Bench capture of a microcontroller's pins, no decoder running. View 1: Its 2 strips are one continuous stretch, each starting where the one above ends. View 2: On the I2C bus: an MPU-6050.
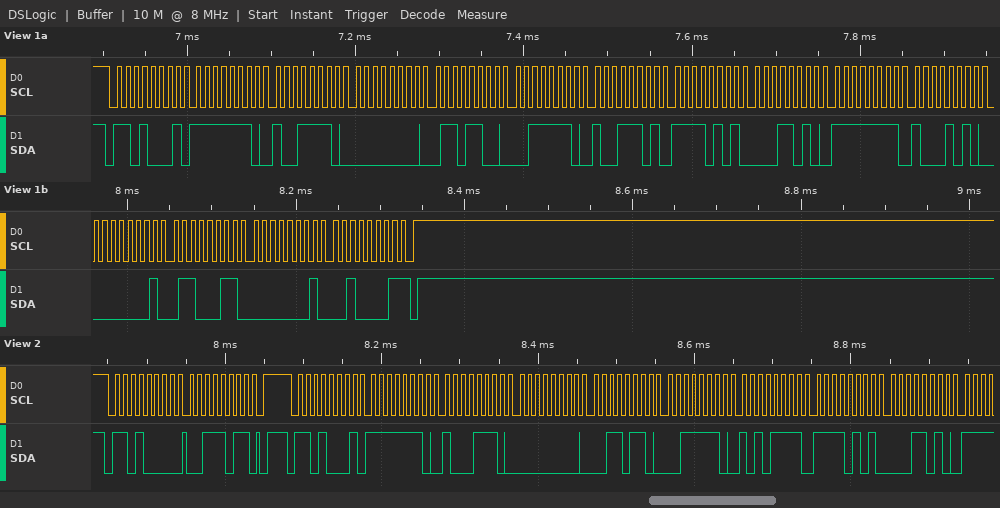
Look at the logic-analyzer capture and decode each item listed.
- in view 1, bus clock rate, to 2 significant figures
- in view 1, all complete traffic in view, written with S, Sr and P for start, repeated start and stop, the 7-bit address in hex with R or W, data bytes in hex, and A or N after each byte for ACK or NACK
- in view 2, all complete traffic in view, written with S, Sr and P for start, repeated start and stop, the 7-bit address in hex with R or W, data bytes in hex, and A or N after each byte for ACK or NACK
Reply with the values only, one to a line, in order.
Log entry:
100 kHz
S 68R A FE A 9E A 00 A 6C A 3E A 9D A F5 A 1A A FF A 8A A 01 A 63 A 01 A 21 N P
S 68W A 3B A P S 68R A FE A 8E A 00 A 36 A 3E A AF A F5 A 1A A
